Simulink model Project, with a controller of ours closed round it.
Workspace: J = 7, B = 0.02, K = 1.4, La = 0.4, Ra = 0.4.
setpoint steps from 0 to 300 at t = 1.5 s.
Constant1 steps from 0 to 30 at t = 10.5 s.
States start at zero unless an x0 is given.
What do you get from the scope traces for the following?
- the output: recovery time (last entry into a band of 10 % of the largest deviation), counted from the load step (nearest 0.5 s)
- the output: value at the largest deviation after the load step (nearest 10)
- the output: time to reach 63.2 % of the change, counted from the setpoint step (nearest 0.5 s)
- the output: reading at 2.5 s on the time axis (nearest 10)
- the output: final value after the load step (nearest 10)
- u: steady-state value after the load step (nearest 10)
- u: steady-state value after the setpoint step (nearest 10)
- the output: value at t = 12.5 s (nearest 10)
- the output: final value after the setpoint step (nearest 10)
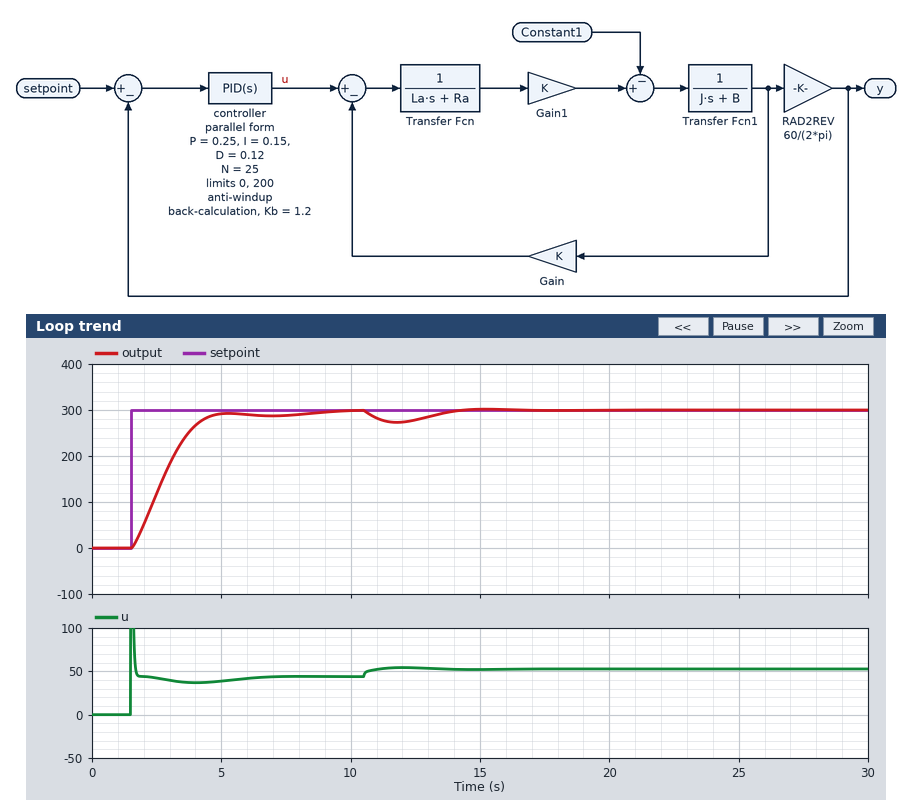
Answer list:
3.5 s
270
1.5 s
120
300
50
40
280
300
